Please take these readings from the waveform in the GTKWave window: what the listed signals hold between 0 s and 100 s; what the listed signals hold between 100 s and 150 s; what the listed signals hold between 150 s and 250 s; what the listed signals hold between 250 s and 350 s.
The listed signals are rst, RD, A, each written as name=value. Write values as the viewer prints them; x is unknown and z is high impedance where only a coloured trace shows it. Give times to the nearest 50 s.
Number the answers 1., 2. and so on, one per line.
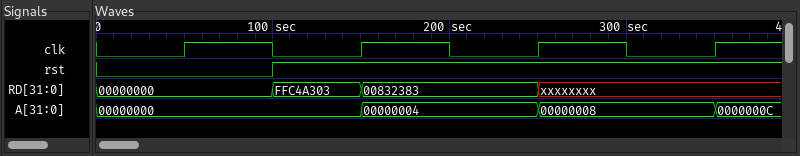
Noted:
1. rst=0, RD=00000000, A=00000000
2. rst=1, RD=FFC4A303, A=00000000
3. rst=1, RD=00832383, A=00000004
4. rst=1, RD=xxxxxxxx, A=00000008
